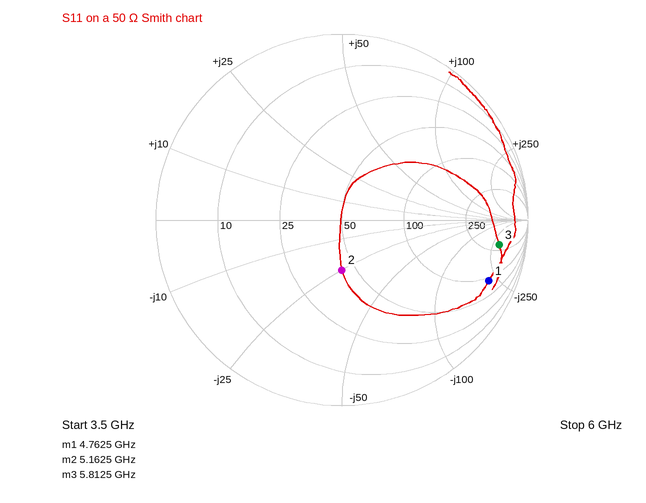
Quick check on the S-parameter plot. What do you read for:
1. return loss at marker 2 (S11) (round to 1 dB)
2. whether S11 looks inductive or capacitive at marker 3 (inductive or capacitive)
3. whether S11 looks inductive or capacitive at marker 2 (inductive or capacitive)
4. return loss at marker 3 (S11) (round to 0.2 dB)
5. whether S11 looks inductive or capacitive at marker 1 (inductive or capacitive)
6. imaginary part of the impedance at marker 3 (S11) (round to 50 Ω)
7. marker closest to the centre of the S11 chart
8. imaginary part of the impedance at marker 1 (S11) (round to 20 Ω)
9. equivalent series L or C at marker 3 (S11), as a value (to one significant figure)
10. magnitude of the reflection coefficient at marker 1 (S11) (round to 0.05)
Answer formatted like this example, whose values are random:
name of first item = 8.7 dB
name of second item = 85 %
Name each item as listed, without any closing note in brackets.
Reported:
return loss at marker 2 (S11) = 11 dB
whether S11 looks inductive or capacitive at marker 3 = capacitive
whether S11 looks inductive or capacitive at marker 2 = capacitive
return loss at marker 3 (S11) = 1.4 dB
whether S11 looks inductive or capacitive at marker 1 = capacitive
imaginary part of the impedance at marker 3 (S11) = -300 Ω
marker closest to the centre of the S11 chart = marker 2
imaginary part of the impedance at marker 1 (S11) = -220 Ω
equivalent series L or C at marker 3 (S11), as a value = 90 fF
magnitude of the reflection coefficient at marker 1 (S11) = 0.85
